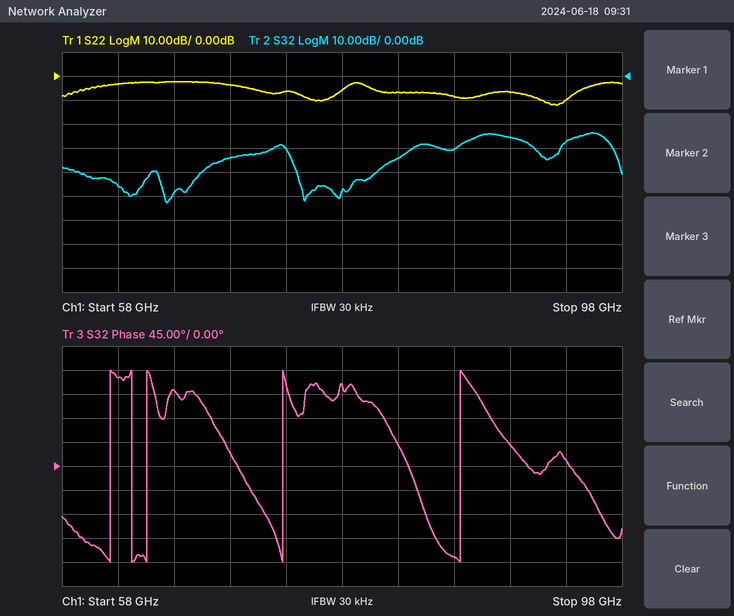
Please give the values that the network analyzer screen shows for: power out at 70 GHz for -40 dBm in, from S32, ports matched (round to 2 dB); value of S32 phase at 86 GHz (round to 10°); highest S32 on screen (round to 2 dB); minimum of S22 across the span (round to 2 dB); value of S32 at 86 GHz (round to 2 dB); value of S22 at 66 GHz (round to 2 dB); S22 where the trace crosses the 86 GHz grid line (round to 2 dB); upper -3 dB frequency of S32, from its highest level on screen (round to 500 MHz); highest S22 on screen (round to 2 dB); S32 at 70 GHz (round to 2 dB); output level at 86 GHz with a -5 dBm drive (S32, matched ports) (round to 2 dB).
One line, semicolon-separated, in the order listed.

-74 dBm; -170°; -24 dB; -12 dB; -30 dB; -2 dB; -8 dB; 97.0 GHz; -2 dB; -34 dB; -36 dBm
